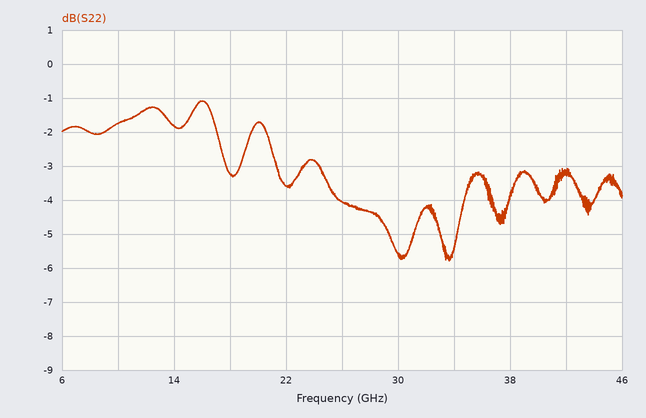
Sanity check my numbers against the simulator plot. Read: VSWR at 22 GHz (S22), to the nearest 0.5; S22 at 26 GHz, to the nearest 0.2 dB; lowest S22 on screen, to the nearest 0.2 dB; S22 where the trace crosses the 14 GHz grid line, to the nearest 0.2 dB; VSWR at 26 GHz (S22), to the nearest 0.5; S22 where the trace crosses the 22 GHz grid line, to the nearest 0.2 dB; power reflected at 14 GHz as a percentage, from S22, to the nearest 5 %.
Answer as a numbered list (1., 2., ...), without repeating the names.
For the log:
1. 5.0
2. -4.0 dB
3. -5.8 dB
4. -1.8 dB
5. 4.5
6. -3.6 dB
7. 65 %
